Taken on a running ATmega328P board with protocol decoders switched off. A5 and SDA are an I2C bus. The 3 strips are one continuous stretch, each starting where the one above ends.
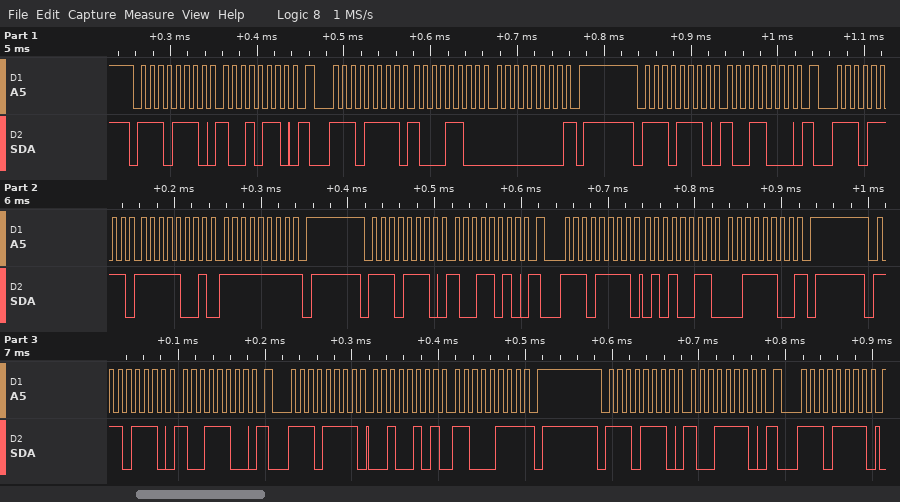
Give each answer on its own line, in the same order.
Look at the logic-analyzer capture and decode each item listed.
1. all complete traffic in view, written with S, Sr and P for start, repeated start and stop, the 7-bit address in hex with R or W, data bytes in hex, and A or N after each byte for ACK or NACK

S 77W A 96 A Sr 77R A 8C A 00 N P S 77W A 98 A Sr 77R A F9 A FF N P S 77W A 9A A Sr 77R A 53 A 3C N P S 77W A 9C A Sr 77R A 25 A C7 N P S 77W A 9E A Sr 77R A
